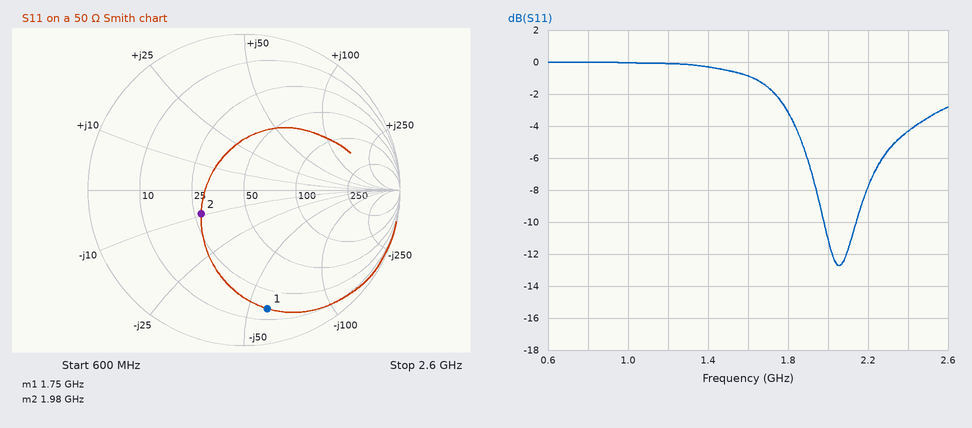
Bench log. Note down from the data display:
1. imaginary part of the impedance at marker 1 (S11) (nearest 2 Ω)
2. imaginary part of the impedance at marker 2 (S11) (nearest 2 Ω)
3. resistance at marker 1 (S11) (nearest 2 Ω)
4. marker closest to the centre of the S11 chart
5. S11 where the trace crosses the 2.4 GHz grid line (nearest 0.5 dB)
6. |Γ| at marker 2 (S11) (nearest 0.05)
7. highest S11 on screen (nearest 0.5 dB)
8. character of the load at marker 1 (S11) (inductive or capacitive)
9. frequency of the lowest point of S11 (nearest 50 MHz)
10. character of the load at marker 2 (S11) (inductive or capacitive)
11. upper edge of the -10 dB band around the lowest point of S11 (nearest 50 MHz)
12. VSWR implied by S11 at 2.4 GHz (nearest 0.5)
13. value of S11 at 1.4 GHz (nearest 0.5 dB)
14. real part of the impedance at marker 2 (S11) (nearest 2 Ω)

-58 Ω
-10 Ω
16 Ω
marker 2
-4.5 dB
0.30
0.0 dB
capacitive
2.05 GHz
capacitive
2.15 GHz
4.0
-0.5 dB
28 Ω
